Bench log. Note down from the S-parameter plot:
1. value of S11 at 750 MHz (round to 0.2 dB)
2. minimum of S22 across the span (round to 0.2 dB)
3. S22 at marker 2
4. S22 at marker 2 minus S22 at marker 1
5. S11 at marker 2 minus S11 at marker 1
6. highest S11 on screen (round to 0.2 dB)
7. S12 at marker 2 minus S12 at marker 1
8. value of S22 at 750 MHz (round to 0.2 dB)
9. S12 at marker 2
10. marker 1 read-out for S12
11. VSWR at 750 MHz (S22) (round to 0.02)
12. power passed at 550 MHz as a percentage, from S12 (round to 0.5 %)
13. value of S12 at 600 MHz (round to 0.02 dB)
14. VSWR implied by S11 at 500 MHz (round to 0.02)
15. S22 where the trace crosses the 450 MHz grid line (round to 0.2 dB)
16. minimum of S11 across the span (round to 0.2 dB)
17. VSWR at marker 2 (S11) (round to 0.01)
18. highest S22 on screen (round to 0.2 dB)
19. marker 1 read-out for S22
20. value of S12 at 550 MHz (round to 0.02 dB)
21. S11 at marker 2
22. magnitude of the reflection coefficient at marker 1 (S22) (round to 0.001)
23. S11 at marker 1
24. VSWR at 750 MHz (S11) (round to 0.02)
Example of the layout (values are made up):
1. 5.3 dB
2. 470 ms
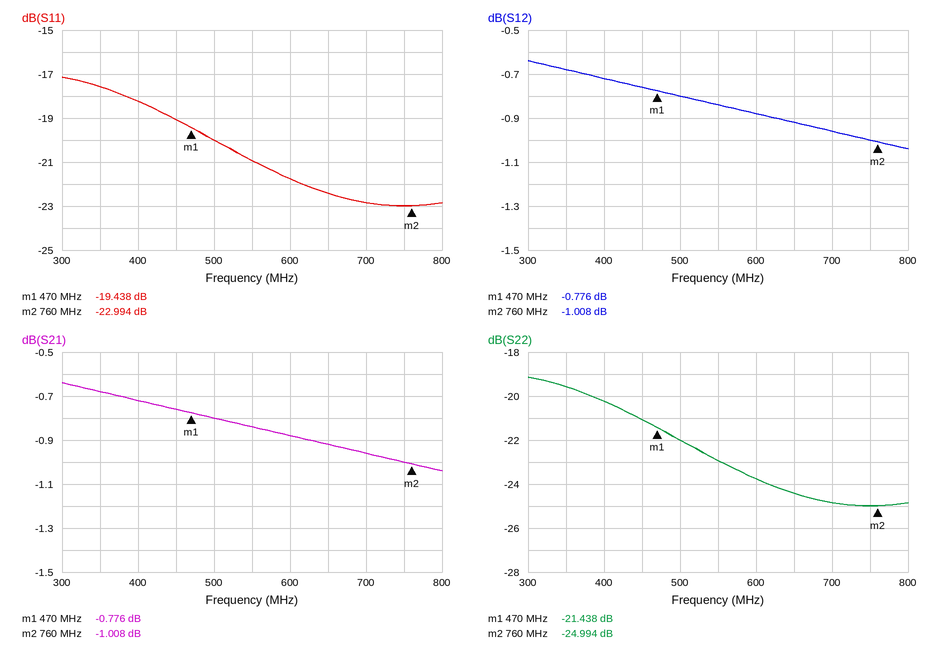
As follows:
1. -23.0 dB
2. -25.0 dB
3. -24.994 dB
4. -3.556 dB
5. -3.556 dB
6. -17.2 dB
7. -0.232 dB
8. -25.0 dB
9. -1.008 dB
10. -0.776 dB
11. 1.12
12. 82.5 %
13. -0.88 dB
14. 1.22
15. -21.0 dB
16. -23.0 dB
17. 1.15
18. -19.2 dB
19. -21.438 dB
20. -0.84 dB
21. -22.994 dB
22. 0.085
23. -19.438 dB
24. 1.16
